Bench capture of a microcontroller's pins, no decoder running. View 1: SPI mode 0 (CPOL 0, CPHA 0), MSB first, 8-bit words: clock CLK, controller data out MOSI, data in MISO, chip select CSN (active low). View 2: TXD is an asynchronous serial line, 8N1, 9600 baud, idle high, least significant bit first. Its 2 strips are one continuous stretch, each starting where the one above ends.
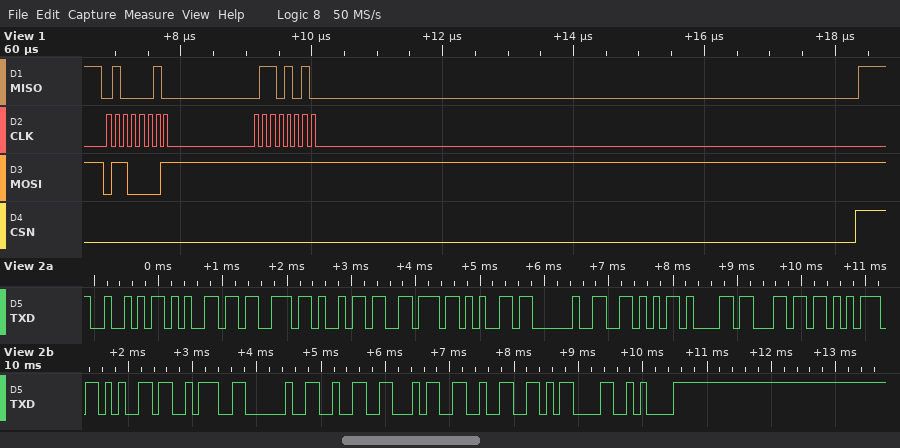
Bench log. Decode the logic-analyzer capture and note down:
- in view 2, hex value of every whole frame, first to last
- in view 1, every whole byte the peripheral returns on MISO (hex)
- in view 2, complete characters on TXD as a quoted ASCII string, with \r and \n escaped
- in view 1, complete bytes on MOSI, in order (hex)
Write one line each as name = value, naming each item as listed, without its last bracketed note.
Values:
in view 2, hex value of every whole frame, first to last = 52 65 73 69 76 65 20 56 61 6C 75 65 3A 20 32 34 32 0D 0A
in view 1, every whole byte the peripheral returns on MISO = 42 6A
in view 2, complete characters on TXD as a quoted ASCII string, with \r and \n escaped = "Resive Value: 242\r\n"
in view 1, complete bytes on MOSI, in order = 61 FF
